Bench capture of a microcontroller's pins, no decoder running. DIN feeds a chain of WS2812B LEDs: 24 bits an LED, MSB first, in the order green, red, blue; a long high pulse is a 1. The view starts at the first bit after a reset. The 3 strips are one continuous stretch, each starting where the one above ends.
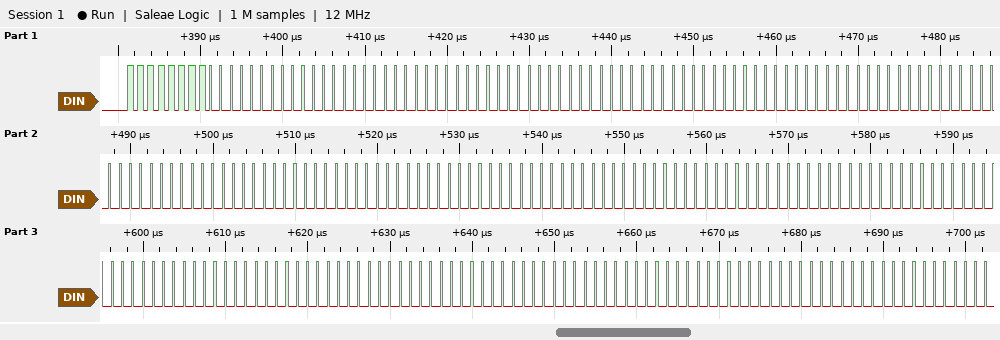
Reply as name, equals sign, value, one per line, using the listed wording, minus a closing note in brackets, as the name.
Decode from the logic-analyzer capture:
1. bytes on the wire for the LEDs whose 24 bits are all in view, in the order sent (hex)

bytes on the wire for the LEDs whose 24 bits are all in view, in the order sent = FF 00 00 00 00 00 00 00 00 00 00 00 00 00 00 00 00 00 00 00 00 00 00 00 00 00 00 00 00 00
